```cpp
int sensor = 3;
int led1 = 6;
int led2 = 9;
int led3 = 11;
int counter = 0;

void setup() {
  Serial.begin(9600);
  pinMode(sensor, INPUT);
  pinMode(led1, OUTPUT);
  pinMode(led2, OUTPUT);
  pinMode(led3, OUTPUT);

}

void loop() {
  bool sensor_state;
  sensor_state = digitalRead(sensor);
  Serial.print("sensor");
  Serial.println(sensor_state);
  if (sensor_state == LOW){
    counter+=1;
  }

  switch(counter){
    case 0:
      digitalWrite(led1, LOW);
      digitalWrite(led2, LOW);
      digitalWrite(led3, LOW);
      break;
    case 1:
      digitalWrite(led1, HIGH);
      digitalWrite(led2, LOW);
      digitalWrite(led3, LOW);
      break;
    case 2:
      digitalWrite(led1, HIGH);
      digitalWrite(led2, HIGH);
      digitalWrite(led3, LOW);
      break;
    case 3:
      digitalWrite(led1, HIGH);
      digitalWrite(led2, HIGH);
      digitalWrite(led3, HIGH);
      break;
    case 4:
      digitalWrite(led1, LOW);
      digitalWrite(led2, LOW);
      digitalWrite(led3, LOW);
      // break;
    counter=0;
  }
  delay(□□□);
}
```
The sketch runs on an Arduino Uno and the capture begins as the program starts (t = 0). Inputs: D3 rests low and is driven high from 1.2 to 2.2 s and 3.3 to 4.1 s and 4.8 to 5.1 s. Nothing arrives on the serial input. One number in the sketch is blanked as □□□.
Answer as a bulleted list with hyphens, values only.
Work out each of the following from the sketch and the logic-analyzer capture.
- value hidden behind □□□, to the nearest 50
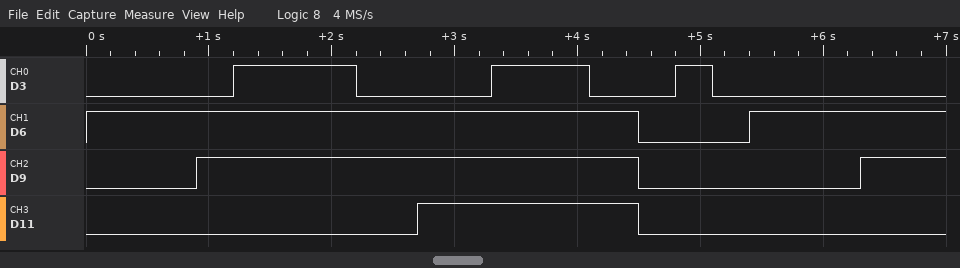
- 900
